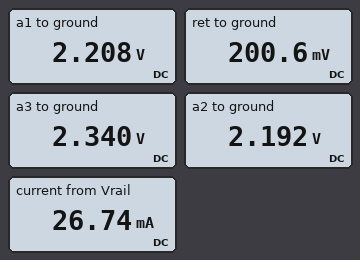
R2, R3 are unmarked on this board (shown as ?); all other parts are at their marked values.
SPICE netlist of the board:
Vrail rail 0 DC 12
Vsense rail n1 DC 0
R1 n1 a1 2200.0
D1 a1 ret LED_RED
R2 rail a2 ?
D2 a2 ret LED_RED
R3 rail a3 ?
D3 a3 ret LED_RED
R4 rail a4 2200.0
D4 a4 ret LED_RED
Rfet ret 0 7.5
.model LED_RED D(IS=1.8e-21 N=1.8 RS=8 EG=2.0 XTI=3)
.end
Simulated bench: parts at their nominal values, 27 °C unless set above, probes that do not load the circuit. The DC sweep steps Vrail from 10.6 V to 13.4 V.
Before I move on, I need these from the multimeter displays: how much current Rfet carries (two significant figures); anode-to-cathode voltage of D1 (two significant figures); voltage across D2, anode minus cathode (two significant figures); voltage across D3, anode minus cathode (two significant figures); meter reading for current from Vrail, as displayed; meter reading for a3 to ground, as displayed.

27 mA
2.0 V
2.0 V
2.1 V
26.74 mA
2.340 V
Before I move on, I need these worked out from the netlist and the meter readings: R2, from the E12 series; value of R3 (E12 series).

2.7 kΩ
680 Ω
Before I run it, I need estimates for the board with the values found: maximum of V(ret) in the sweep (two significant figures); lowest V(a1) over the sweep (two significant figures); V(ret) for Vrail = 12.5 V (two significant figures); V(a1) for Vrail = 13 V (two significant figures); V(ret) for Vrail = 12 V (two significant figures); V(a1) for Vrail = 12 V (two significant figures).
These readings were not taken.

230 mV
2.2 V
210 mV
2.2 V
200 mV
2.2 V
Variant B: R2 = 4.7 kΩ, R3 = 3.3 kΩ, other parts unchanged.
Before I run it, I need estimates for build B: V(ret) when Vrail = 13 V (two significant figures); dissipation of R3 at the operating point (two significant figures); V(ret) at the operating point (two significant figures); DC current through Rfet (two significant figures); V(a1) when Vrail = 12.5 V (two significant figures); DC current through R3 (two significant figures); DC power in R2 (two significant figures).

120 mV
30 mW
110 mV
14 mA
2.1 V
3.0 mA
21 mW
